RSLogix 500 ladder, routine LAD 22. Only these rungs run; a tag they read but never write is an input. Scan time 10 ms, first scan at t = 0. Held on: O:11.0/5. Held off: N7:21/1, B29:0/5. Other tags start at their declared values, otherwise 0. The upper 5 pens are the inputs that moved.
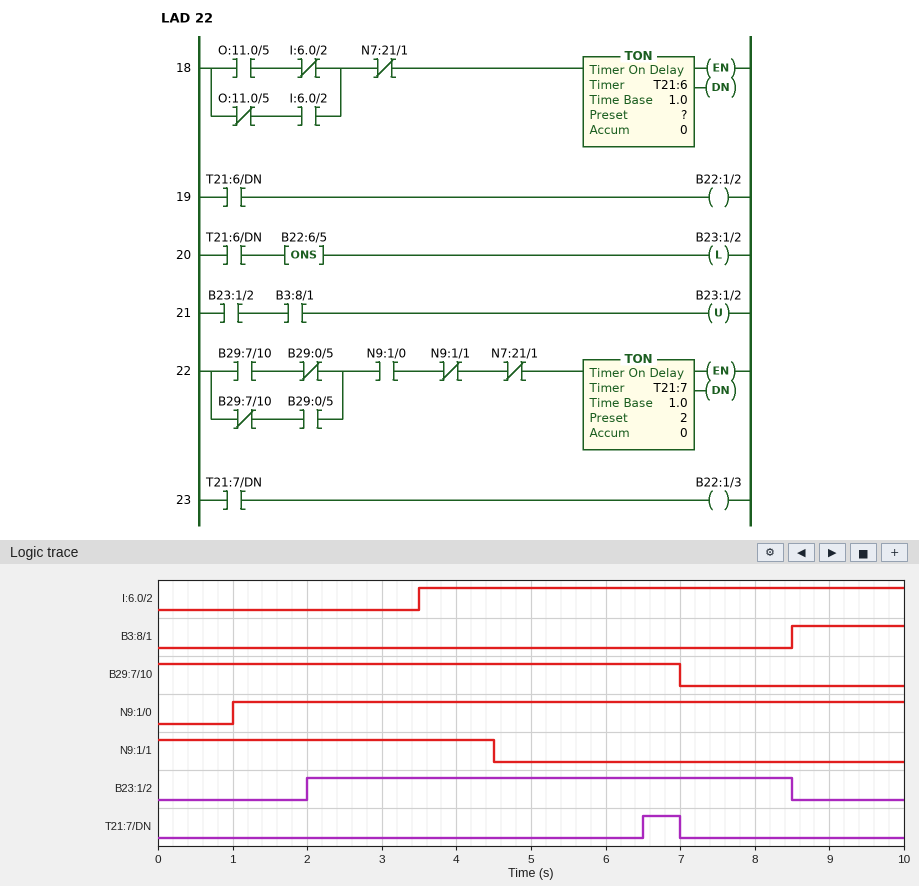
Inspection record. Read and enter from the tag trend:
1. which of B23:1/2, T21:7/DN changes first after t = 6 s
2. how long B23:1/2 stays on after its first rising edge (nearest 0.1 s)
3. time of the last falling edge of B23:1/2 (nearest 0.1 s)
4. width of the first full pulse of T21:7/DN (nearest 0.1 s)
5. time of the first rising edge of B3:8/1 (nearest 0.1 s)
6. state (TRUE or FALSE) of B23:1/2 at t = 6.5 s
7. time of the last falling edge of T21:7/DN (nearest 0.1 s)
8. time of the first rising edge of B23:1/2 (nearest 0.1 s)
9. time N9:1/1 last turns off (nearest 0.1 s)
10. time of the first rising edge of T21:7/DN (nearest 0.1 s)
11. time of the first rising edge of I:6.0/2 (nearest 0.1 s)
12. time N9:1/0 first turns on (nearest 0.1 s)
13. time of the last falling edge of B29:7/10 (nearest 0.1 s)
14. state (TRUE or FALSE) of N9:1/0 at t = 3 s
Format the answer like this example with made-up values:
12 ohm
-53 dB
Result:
T21:7/DN
6.5 s
8.5 s
0.5 s
8.5 s
TRUE
7.0 s
2.0 s
4.5 s
6.5 s
3.5 s
1.0 s
7.0 s
TRUE
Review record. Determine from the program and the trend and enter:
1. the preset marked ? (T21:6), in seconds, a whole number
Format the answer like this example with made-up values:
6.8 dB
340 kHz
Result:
2 s
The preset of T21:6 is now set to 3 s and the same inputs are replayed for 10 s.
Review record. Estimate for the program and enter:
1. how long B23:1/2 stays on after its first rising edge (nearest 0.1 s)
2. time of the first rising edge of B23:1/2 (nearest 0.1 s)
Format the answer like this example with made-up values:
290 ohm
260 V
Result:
5.5 s
3.0 s
